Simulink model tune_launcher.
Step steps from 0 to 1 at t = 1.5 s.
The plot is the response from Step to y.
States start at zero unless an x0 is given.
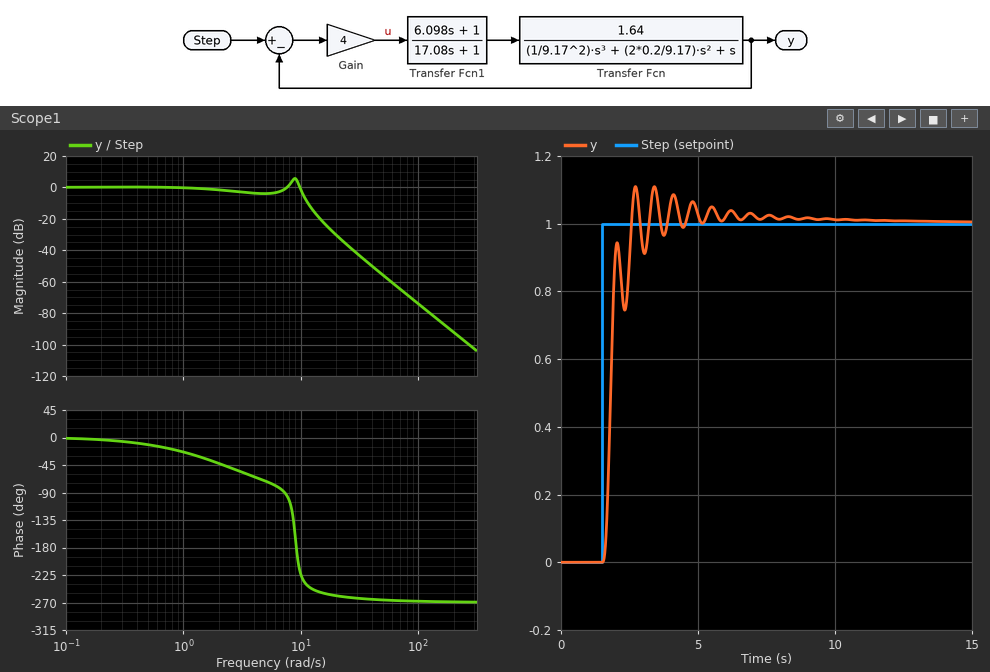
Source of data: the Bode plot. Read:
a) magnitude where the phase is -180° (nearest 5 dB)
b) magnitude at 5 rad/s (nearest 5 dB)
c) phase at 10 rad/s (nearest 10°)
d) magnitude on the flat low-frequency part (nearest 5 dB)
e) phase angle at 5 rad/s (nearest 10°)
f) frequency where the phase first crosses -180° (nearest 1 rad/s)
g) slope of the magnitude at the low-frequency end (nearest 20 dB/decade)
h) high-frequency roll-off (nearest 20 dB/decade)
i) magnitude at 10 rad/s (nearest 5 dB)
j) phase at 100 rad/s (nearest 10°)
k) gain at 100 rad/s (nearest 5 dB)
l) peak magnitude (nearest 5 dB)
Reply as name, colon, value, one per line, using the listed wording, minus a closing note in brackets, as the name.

magnitude where the phase is -180°: 5 dB
magnitude at 5 rad/s: -5 dB
phase at 10 rad/s: -220°
magnitude on the flat low-frequency part: 0 dB
phase angle at 5 rad/s: -70°
frequency where the phase first crosses -180°: 9 rad/s
slope of the magnitude at the low-frequency end: 0 dB/decade
high-frequency roll-off: -60 dB/decade
magnitude at 10 rad/s: 0 dB
phase at 100 rad/s: -270°
gain at 100 rad/s: -75 dB
peak magnitude: 5 dB
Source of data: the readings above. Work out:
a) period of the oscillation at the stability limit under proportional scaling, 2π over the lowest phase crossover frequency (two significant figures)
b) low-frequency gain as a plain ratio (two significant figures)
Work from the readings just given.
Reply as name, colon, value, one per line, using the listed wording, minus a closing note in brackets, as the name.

period of the oscillation at the stability limit under proportional scaling, 2π over the lowest phase crossover frequency: 0.70 s
low-frequency gain as a plain ratio: 1.0
